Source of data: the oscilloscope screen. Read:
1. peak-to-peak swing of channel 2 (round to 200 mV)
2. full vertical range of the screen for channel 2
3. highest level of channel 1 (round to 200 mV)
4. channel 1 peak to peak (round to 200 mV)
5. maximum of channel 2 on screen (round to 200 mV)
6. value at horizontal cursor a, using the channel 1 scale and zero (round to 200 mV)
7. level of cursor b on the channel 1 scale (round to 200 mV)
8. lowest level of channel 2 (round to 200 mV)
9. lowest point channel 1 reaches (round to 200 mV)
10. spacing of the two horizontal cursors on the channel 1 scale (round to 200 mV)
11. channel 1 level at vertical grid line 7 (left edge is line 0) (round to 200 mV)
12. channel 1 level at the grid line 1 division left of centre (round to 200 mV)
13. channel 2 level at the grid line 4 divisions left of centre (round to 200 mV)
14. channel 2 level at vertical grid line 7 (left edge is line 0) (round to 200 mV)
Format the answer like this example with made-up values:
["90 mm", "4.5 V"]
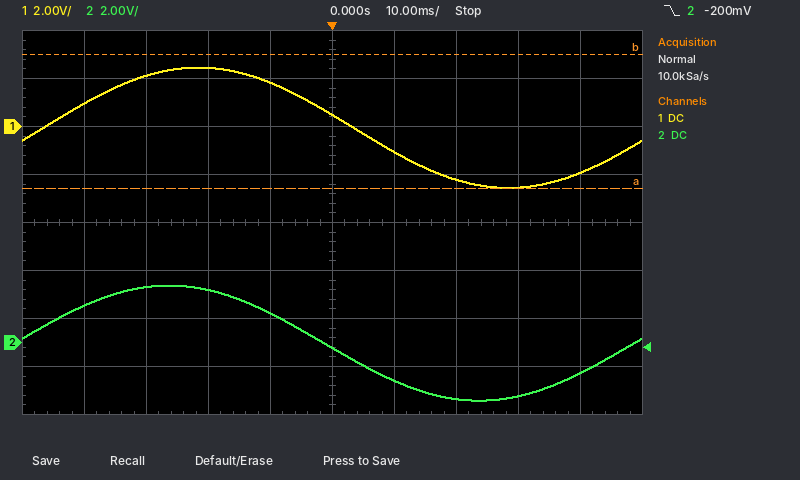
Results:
["4.8 V", "16 V", "2.4 V", "5.0 V", "2.4 V", "-2.6 V", "3.0 V", "-2.4 V", "-2.6 V", "5.6 V", "-2.2 V", "1.8 V", "1.6 V", "-2.4 V"]
